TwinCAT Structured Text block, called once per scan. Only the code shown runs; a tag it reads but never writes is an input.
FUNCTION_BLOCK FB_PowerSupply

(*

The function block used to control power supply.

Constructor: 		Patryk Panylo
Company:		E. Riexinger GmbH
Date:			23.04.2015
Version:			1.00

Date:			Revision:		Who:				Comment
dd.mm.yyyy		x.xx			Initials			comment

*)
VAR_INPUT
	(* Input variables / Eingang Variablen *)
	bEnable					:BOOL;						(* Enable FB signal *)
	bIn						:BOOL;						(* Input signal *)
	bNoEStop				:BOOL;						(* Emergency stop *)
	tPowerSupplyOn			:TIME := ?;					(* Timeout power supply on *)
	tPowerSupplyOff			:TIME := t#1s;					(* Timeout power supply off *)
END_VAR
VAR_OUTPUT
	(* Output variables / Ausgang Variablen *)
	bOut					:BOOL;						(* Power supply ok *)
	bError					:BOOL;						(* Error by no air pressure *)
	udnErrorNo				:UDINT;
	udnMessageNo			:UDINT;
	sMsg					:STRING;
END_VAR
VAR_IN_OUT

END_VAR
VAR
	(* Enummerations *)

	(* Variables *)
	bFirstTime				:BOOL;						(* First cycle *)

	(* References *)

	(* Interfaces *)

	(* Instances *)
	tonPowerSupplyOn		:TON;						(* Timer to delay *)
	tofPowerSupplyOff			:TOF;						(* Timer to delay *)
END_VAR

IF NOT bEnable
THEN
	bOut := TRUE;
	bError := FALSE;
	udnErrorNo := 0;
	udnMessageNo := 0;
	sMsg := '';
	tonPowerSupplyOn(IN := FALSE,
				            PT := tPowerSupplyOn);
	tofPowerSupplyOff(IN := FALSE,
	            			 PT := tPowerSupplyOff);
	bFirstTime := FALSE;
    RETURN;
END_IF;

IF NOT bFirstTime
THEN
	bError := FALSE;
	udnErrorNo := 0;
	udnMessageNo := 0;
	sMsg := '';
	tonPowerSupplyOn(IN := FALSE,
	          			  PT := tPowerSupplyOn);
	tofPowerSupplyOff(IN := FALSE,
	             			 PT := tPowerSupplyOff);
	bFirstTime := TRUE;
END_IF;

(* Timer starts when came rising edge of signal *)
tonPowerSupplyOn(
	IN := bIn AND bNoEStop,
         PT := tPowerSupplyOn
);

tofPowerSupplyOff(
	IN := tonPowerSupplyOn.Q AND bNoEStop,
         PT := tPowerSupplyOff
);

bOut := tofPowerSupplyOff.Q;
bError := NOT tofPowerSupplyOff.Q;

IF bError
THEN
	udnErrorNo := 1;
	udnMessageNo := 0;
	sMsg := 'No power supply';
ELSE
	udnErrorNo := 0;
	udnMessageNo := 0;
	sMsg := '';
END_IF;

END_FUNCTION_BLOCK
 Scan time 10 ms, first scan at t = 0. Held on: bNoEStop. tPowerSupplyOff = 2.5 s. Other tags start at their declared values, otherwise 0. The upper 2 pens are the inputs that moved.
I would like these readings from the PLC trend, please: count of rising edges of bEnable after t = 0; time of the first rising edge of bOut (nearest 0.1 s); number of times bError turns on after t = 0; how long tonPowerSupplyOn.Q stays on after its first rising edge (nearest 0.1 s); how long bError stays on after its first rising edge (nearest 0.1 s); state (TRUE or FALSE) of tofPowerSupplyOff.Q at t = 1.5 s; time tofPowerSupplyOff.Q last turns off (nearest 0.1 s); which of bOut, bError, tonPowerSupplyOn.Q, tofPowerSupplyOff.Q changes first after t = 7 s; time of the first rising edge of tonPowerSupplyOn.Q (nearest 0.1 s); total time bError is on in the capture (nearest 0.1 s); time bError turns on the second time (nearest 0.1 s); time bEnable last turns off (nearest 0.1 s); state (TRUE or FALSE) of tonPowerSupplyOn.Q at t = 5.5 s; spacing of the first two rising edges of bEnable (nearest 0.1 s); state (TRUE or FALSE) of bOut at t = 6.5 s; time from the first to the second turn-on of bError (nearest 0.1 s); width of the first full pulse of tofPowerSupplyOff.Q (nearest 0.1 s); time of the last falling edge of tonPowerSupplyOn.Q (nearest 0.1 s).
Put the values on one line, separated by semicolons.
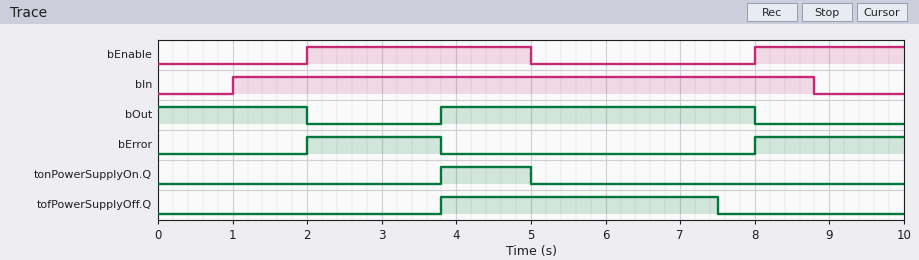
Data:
2; 3.8 s; 2; 1.2 s; 1.8 s; FALSE; 7.5 s; tofPowerSupplyOff.Q; 3.8 s; 3.8 s; 8.0 s; 5.0 s; FALSE; 6.0 s; TRUE; 6.0 s; 3.7 s; 5.0 s
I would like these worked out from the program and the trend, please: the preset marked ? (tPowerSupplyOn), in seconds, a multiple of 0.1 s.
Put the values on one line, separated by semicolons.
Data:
1.8 s
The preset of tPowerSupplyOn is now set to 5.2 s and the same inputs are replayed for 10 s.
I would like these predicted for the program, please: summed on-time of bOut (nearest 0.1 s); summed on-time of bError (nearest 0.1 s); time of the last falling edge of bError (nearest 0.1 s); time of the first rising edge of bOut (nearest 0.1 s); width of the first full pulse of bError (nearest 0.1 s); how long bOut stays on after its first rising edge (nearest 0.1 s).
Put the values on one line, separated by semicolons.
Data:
5.0 s; 5.0 s; 5.0 s; 5.0 s; 3.0 s; 3.0 s
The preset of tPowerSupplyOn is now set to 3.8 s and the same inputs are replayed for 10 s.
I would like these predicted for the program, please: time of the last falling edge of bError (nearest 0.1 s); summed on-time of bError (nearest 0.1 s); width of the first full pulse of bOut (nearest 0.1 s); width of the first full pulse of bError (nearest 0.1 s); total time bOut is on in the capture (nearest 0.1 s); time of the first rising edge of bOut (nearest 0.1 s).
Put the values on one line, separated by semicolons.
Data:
5.0 s; 5.0 s; 3.0 s; 3.0 s; 5.0 s; 5.0 s
